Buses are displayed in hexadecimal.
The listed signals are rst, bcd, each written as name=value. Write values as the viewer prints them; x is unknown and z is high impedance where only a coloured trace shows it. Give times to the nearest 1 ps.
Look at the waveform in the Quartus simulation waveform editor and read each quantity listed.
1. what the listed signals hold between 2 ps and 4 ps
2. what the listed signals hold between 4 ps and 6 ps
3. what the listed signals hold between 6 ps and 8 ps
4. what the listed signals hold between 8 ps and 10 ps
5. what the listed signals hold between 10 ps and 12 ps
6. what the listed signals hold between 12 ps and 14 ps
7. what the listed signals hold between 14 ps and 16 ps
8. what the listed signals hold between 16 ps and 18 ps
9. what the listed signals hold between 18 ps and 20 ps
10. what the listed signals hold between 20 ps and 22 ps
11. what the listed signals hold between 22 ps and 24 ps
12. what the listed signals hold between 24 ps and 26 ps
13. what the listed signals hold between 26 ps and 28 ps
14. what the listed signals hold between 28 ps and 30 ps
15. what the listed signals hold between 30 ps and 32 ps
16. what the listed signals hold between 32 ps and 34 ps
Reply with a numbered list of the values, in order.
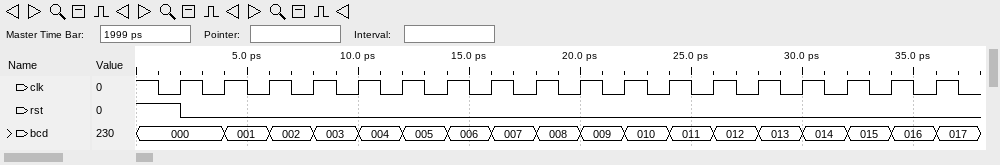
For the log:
1. rst=0, bcd=000
2. rst=0, bcd=001
3. rst=0, bcd=002
4. rst=0, bcd=003
5. rst=0, bcd=004
6. rst=0, bcd=005
7. rst=0, bcd=006
8. rst=0, bcd=007
9. rst=0, bcd=008
10. rst=0, bcd=009
11. rst=0, bcd=010
12. rst=0, bcd=011
13. rst=0, bcd=012
14. rst=0, bcd=013
15. rst=0, bcd=014
16. rst=0, bcd=015
